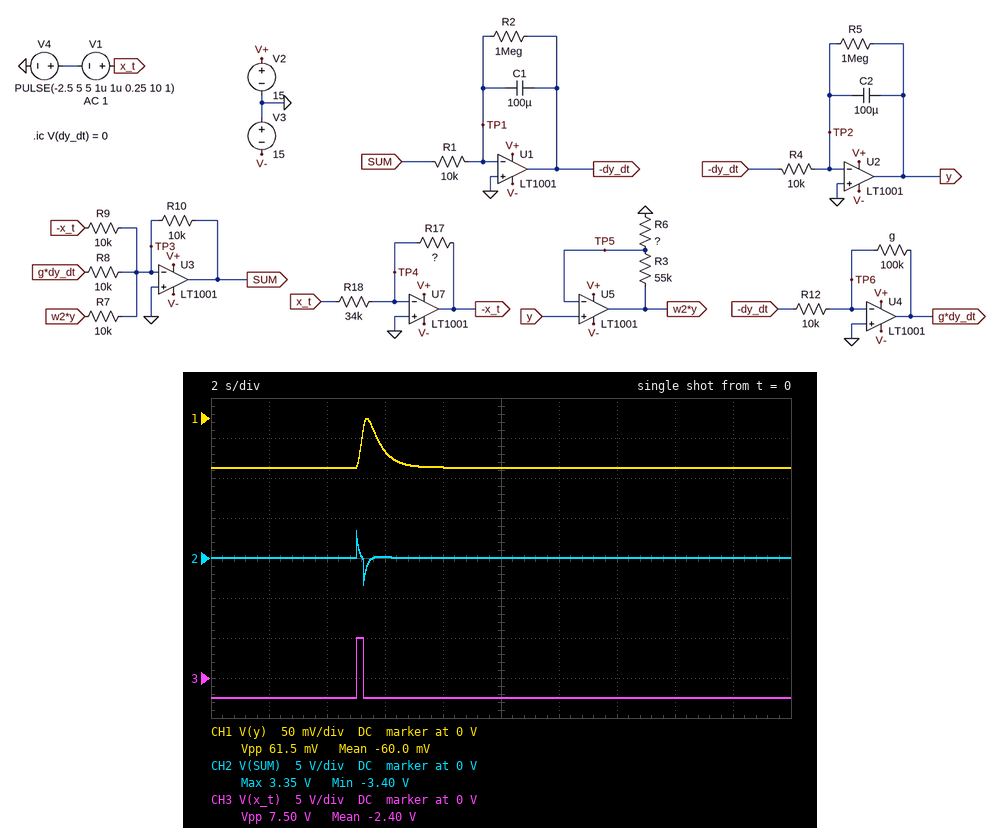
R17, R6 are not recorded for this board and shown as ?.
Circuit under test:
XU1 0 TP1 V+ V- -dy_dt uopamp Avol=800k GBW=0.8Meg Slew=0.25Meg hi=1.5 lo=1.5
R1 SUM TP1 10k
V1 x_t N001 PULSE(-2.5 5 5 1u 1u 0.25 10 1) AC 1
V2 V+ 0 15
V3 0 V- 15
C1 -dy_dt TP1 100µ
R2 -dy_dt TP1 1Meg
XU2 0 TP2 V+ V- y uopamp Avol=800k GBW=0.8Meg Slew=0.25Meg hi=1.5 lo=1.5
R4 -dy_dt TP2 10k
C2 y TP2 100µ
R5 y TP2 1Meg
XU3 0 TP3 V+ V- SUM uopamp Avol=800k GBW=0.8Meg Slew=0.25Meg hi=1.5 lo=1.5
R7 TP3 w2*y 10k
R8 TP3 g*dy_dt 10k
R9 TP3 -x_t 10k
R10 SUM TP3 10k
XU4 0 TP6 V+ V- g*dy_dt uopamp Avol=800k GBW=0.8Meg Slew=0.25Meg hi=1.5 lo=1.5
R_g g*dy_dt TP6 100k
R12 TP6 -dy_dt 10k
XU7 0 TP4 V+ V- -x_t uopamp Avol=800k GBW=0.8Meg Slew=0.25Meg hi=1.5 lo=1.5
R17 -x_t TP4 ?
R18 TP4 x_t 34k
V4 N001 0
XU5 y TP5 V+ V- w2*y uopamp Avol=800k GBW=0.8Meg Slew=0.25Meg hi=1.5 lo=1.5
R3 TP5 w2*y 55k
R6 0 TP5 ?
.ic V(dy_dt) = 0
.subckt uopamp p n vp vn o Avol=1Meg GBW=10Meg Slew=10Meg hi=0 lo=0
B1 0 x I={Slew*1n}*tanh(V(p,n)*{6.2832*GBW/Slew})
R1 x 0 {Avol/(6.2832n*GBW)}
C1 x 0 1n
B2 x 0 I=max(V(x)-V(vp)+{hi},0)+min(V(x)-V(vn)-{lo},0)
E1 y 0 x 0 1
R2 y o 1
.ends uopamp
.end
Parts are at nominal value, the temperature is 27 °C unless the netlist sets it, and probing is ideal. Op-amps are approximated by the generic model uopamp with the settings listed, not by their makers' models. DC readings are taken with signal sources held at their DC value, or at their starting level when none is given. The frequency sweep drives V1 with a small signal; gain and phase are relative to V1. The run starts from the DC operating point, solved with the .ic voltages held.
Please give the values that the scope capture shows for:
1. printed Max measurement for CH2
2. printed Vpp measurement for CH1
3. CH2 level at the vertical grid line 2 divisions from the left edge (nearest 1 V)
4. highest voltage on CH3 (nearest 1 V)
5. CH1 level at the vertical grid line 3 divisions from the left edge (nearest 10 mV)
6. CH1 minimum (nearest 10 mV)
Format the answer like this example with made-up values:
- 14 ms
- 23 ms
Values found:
- 3.35 V
- 61.5 mV
- 0 V
- 5 V
- -40 mV
- -60 mV
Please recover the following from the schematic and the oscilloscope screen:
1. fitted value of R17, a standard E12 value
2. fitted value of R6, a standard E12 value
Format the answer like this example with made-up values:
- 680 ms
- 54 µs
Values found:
- 15 kΩ
- 3.3 kΩ
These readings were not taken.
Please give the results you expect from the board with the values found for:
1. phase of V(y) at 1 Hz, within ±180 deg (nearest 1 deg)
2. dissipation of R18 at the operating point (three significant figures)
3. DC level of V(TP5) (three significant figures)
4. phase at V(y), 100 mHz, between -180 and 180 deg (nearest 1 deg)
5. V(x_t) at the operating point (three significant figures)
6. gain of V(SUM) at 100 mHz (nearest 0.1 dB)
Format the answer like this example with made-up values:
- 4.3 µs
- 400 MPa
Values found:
- -109 deg
- 184 µW
- -62.1 mV
- -20 deg
- -2.50 V
- -40.5 dB
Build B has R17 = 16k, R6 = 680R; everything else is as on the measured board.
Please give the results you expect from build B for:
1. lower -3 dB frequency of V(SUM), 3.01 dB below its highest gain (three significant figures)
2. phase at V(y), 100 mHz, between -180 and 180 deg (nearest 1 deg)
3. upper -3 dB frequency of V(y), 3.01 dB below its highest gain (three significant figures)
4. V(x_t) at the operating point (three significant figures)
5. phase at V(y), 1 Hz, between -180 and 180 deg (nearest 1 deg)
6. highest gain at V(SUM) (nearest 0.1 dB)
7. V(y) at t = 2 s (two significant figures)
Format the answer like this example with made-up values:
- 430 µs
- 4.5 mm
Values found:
- 1.26 Hz
- -4 deg
- 1.65 Hz
- -2.50 V
- -56 deg
- -5.8 dB
- -14 mV
